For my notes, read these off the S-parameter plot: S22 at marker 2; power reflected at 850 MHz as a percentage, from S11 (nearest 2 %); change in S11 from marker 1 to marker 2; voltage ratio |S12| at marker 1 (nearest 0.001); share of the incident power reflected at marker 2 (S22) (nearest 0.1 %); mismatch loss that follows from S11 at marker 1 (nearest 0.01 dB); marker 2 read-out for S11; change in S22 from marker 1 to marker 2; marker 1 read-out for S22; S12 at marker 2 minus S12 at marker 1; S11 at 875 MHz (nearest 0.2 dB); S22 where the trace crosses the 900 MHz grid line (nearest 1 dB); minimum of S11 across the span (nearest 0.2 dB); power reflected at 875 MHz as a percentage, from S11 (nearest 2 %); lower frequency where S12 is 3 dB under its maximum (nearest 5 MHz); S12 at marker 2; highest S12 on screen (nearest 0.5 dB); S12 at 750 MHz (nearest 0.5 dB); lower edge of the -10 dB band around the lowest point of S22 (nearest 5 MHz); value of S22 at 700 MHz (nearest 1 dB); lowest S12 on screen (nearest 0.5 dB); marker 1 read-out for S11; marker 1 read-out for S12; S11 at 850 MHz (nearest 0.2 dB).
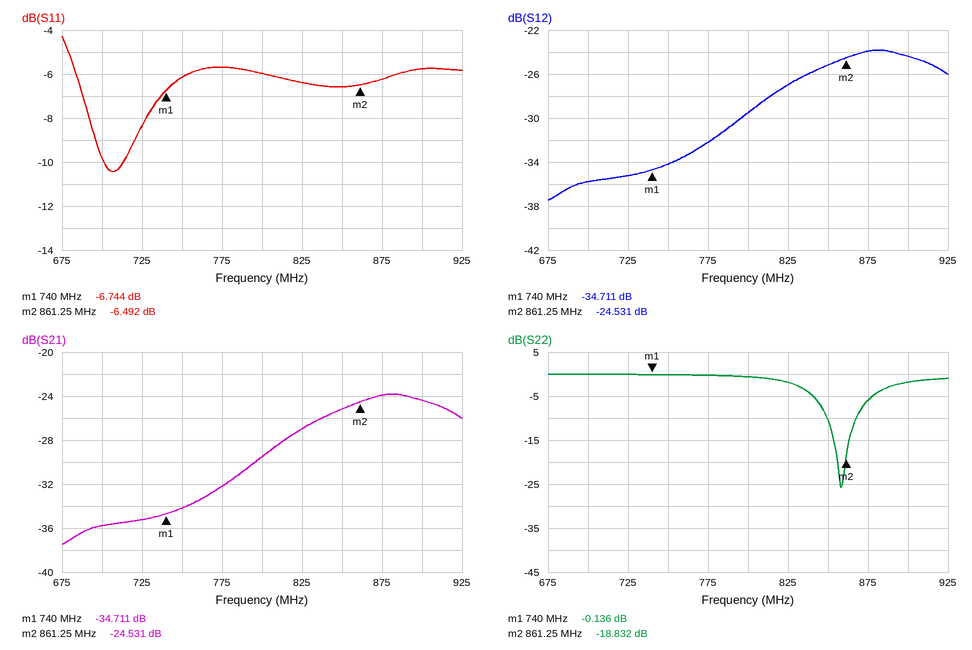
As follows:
-18.832 dB
22 %
0.252 dB
0.018
1.3 %
1.03 dB
-6.492 dB
-18.696 dB
-0.136 dB
10.180 dB
-6.2 dB
-2 dB
-10.4 dB
24 %
825 MHz
-24.531 dB
-24.0 dB
-34.0 dB
850 MHz
0 dB
-37.5 dB
-6.744 dB
-34.711 dB
-6.6 dB
